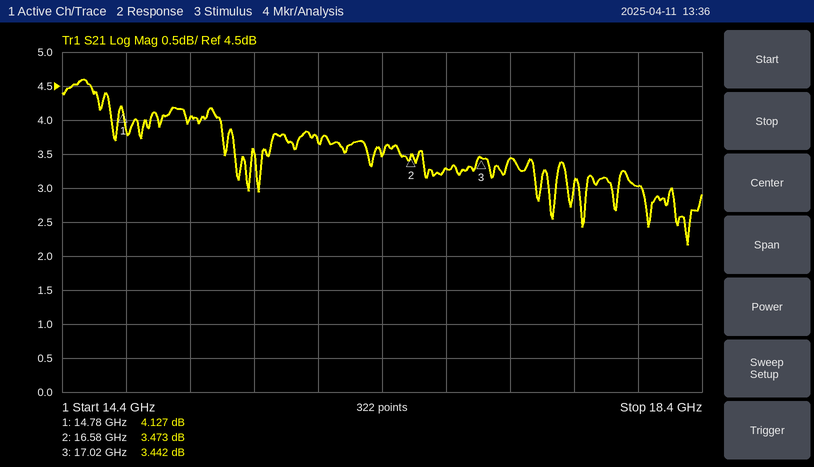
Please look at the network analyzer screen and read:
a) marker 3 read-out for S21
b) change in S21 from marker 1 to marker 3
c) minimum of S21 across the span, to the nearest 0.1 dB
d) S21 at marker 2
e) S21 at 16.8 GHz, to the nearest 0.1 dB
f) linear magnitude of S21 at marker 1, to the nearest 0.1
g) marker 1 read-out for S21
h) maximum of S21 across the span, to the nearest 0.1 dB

3.442 dB
-0.685 dB
2.2 dB
3.473 dB
3.3 dB
1.6
4.127 dB
4.6 dB
